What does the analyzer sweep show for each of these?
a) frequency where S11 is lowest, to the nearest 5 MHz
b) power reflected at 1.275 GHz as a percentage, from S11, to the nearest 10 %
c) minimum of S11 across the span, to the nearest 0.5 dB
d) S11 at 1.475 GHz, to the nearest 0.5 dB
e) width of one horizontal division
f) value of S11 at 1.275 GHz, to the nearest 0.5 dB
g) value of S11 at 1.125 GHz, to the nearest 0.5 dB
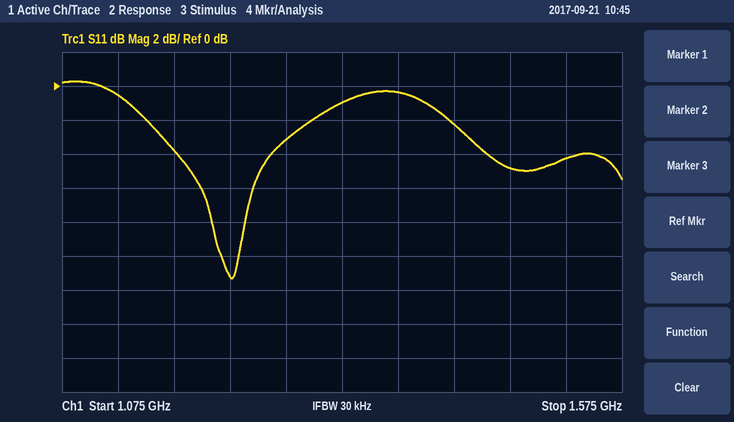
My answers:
1.225 GHz
50 %
-11.5 dB
-5.0 dB
50 MHz
-3.0 dB
-0.5 dB
